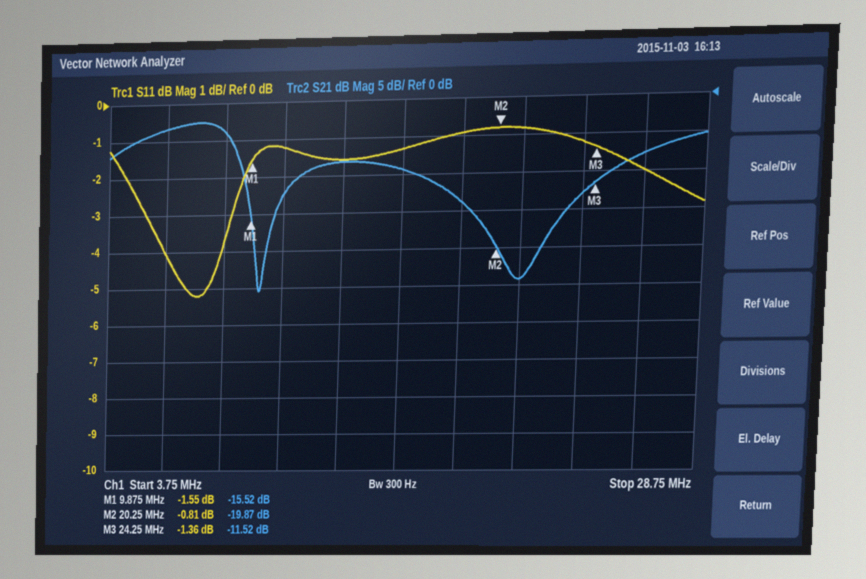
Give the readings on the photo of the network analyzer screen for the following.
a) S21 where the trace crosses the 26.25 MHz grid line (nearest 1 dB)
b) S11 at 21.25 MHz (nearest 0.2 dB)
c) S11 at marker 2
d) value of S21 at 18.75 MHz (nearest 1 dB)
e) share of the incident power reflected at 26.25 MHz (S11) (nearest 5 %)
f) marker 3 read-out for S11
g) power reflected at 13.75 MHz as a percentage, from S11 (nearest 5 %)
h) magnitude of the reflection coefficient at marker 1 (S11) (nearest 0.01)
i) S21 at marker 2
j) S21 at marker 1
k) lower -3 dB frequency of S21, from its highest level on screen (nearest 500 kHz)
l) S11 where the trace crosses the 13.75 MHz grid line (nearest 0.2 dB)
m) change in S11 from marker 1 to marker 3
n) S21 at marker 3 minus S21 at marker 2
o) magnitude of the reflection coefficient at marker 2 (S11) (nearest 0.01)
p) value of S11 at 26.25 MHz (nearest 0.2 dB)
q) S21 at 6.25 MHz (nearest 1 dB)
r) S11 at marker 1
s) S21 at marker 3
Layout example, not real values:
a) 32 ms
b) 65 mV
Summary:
a) -8 dB
b) -0.8 dB
c) -0.81 dB
d) -14 dB
e) 65 %
f) -1.36 dB
g) 70 %
h) 0.84
i) -19.87 dB
j) -15.52 dB
k) 4.5 MHz
l) -1.6 dB
m) 0.19 dB
n) 8.35 dB
o) 0.91
p) -2.0 dB
q) -3 dB
r) -1.55 dB
s) -11.52 dB
